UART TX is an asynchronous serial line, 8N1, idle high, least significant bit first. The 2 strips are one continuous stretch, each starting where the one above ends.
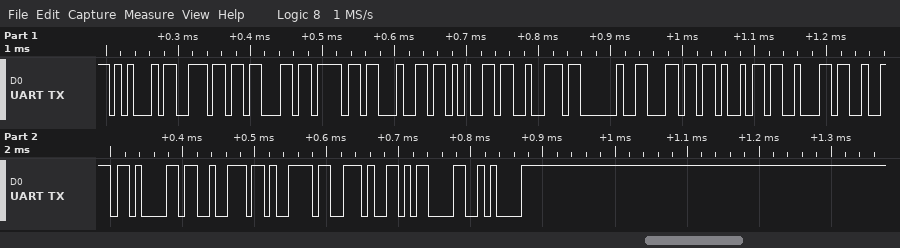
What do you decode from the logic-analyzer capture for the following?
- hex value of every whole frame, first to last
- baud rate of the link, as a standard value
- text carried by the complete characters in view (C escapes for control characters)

0x45 0x6E 0x63 0x6F 0x64 0x65 0x72 0x20 0x6C 0x69 0x62 0x72 0x61 0x72 0x79 0x2E 0x0D 0x0A
115200 baud
"Encoder library.\r\n"
